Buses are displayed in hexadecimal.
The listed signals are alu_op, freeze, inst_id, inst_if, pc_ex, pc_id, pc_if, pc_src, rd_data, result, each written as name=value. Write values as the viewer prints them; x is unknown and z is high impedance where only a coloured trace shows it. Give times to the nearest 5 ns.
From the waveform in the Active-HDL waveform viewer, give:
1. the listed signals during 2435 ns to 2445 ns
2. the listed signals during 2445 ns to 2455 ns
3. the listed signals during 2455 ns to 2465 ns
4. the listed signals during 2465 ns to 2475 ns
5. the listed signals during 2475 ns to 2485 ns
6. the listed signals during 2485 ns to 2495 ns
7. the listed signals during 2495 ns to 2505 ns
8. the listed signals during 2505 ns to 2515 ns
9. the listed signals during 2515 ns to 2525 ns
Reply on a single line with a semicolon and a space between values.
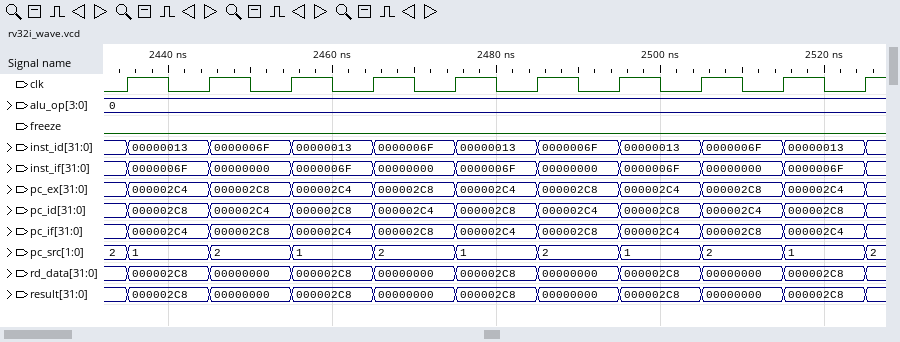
alu_op=0, freeze=0, inst_id=00000013, inst_if=0000006F, pc_ex=000002C4, pc_id=000002C8, pc_if=000002C4, pc_src=1, rd_data=000002C8, result=000002C8; alu_op=0, freeze=0, inst_id=0000006F, inst_if=00000000, pc_ex=000002C8, pc_id=000002C4, pc_if=000002C8, pc_src=2, rd_data=00000000, result=00000000; alu_op=0, freeze=0, inst_id=00000013, inst_if=0000006F, pc_ex=000002C4, pc_id=000002C8, pc_if=000002C4, pc_src=1, rd_data=000002C8, result=000002C8; alu_op=0, freeze=0, inst_id=0000006F, inst_if=00000000, pc_ex=000002C8, pc_id=000002C4, pc_if=000002C8, pc_src=2, rd_data=00000000, result=00000000; alu_op=0, freeze=0, inst_id=00000013, inst_if=0000006F, pc_ex=000002C4, pc_id=000002C8, pc_if=000002C4, pc_src=1, rd_data=000002C8, result=000002C8; alu_op=0, freeze=0, inst_id=0000006F, inst_if=00000000, pc_ex=000002C8, pc_id=000002C4, pc_if=000002C8, pc_src=2, rd_data=00000000, result=00000000; alu_op=0, freeze=0, inst_id=00000013, inst_if=0000006F, pc_ex=000002C4, pc_id=000002C8, pc_if=000002C4, pc_src=1, rd_data=000002C8, result=000002C8; alu_op=0, freeze=0, inst_id=0000006F, inst_if=00000000, pc_ex=000002C8, pc_id=000002C4, pc_if=000002C8, pc_src=2, rd_data=00000000, result=00000000; alu_op=0, freeze=0, inst_id=00000013, inst_if=0000006F, pc_ex=000002C4, pc_id=000002C8, pc_if=000002C4, pc_src=1, rd_data=000002C8, result=000002C8
